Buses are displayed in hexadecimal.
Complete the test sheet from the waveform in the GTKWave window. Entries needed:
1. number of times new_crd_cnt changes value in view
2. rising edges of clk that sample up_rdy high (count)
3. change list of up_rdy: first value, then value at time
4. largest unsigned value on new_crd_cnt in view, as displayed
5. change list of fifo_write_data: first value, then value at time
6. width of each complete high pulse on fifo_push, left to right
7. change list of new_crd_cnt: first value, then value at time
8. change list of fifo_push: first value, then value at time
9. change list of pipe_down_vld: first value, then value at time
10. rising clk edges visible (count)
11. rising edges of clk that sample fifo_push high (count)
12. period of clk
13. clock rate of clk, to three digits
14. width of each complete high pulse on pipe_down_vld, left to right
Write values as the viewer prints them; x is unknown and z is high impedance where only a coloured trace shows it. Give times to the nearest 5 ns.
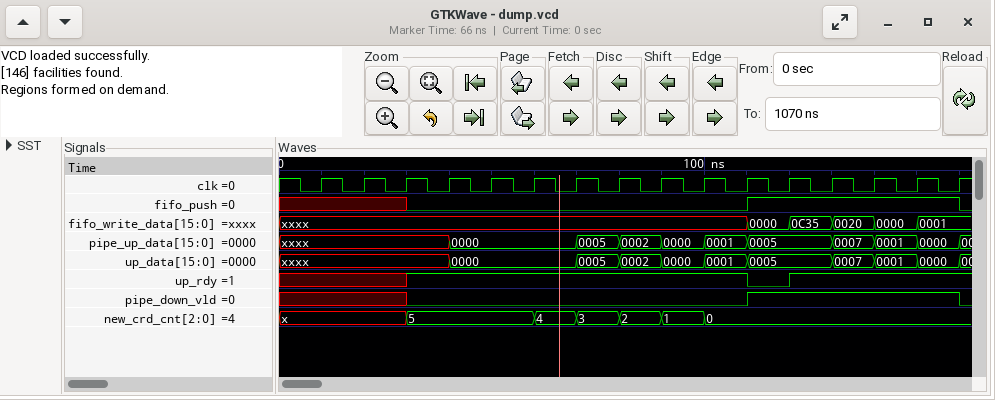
6
12
x, 1 at 30 ns, 0 at 110 ns, 1 at 120 ns
5
xxxx, 0000 at 110 ns, 0C35 at 120 ns, 0020 at 130 ns, 0000 at 140 ns, 0001 at 150 ns
50 ns
x, 5 at 30 ns, 4 at 60 ns, 3 at 70 ns, 2 at 80 ns, 1 at 90 ns, 0 at 100 ns
x, 0 at 30 ns, 1 at 110 ns, 0 at 160 ns
x, 0 at 30 ns, 1 at 110 ns, 0 at 160 ns
16
5
10 ns
100 MHz
50 ns
